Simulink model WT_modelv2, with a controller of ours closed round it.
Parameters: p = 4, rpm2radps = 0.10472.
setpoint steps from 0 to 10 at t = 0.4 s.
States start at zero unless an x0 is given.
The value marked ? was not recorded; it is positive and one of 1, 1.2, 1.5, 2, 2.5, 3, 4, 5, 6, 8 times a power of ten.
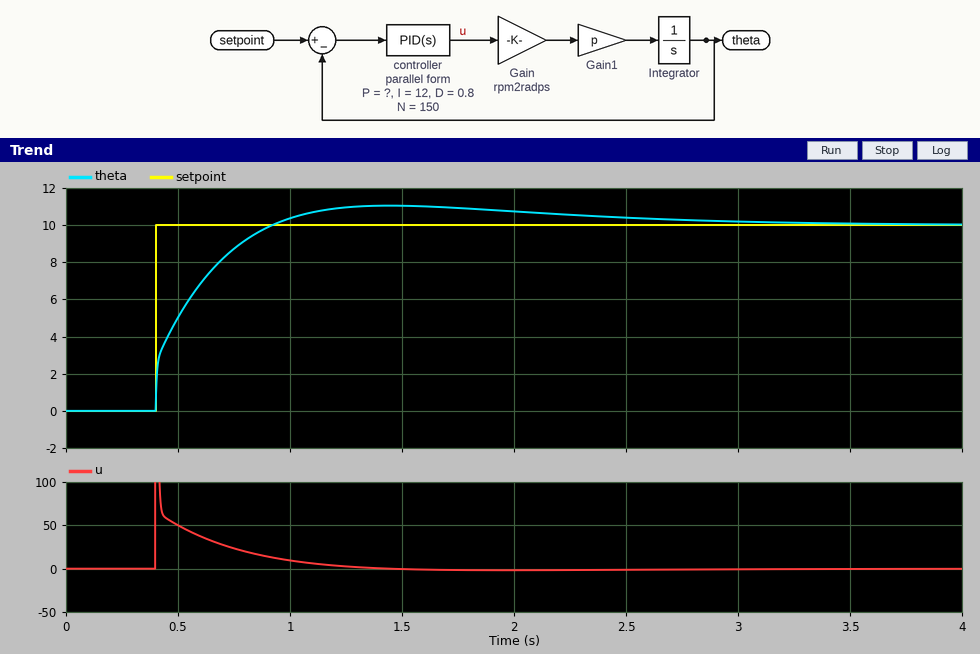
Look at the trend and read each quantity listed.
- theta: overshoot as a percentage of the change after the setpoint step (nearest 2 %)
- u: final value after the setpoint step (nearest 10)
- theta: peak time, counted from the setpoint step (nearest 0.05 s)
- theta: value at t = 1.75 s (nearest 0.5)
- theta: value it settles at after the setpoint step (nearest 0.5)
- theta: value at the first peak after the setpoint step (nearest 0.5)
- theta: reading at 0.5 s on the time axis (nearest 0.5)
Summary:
10 %
0
1.05 s
11.0
10.0
11.0
5.0
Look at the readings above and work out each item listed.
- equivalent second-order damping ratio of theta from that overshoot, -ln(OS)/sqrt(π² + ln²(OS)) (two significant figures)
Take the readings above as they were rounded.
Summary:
0.59
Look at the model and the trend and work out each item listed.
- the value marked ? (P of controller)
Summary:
12
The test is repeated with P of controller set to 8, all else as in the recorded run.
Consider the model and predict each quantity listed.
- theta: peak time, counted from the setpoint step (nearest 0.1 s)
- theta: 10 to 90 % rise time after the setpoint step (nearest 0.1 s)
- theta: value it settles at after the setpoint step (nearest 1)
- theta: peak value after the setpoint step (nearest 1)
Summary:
1.2 s
0.5 s
10
12
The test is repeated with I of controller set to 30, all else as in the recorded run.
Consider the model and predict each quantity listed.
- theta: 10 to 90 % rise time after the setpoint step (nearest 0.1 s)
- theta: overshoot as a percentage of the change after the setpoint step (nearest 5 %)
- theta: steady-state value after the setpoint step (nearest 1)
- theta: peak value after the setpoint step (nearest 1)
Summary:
0.3 s
20 %
10
12
